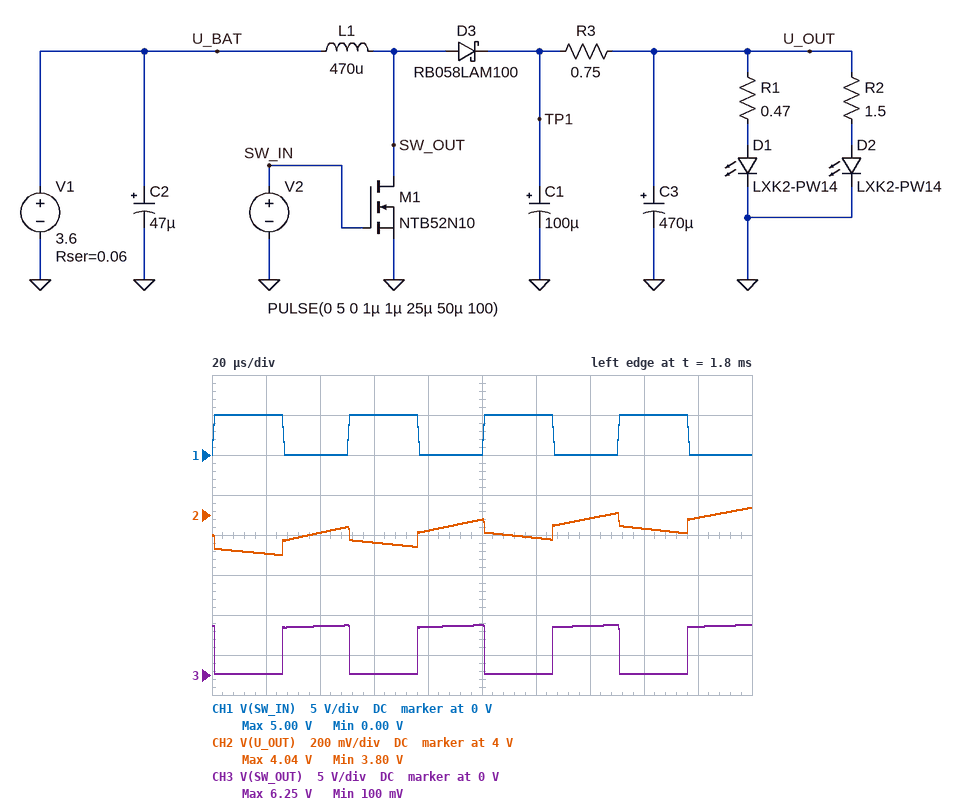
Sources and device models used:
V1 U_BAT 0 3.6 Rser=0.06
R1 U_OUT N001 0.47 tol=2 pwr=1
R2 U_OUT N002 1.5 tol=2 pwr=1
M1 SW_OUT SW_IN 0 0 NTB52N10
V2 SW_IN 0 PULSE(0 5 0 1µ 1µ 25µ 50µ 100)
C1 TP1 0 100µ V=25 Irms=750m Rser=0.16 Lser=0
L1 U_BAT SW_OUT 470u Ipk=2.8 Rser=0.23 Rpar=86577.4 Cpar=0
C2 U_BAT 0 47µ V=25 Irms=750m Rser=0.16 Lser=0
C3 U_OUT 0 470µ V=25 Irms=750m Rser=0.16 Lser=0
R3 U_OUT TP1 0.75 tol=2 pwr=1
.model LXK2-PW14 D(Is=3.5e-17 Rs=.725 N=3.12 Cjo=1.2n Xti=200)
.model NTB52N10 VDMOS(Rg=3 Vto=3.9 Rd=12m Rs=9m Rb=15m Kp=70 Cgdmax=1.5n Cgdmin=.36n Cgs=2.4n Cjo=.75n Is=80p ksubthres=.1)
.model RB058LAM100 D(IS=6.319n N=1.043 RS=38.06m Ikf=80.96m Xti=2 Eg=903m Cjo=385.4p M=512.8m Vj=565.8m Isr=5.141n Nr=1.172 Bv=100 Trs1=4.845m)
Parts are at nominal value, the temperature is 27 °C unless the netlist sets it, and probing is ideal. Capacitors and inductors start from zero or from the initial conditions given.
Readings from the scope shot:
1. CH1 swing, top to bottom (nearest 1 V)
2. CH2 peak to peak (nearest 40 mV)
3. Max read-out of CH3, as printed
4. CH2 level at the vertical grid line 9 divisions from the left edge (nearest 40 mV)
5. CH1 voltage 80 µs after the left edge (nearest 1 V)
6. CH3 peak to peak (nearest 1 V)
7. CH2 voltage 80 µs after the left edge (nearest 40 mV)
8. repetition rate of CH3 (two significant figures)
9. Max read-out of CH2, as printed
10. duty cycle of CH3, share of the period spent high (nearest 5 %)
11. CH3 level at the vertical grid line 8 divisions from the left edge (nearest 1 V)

5 V
240 mV
6.25 V
4.00 V
0 V
6 V
3.92 V
20 kHz
4.04 V
50 %
0 V
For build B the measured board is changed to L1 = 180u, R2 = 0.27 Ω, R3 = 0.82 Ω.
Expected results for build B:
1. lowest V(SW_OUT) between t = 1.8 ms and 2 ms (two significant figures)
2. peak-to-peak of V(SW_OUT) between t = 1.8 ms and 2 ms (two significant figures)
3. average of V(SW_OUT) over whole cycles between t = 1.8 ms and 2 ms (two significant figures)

86 mV
5.8 V
2.9 V
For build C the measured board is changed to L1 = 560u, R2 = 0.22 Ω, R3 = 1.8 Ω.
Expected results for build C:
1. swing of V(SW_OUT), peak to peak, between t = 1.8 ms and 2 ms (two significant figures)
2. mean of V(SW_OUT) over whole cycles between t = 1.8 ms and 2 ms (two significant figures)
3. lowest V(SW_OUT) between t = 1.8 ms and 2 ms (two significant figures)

6.7 V
3.3 V
90 mV
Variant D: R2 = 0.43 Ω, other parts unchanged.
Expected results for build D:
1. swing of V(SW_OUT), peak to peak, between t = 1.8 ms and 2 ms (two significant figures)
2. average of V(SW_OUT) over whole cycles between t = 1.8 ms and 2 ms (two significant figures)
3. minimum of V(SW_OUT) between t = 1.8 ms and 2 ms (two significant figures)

6.0 V
3.0 V
110 mV
